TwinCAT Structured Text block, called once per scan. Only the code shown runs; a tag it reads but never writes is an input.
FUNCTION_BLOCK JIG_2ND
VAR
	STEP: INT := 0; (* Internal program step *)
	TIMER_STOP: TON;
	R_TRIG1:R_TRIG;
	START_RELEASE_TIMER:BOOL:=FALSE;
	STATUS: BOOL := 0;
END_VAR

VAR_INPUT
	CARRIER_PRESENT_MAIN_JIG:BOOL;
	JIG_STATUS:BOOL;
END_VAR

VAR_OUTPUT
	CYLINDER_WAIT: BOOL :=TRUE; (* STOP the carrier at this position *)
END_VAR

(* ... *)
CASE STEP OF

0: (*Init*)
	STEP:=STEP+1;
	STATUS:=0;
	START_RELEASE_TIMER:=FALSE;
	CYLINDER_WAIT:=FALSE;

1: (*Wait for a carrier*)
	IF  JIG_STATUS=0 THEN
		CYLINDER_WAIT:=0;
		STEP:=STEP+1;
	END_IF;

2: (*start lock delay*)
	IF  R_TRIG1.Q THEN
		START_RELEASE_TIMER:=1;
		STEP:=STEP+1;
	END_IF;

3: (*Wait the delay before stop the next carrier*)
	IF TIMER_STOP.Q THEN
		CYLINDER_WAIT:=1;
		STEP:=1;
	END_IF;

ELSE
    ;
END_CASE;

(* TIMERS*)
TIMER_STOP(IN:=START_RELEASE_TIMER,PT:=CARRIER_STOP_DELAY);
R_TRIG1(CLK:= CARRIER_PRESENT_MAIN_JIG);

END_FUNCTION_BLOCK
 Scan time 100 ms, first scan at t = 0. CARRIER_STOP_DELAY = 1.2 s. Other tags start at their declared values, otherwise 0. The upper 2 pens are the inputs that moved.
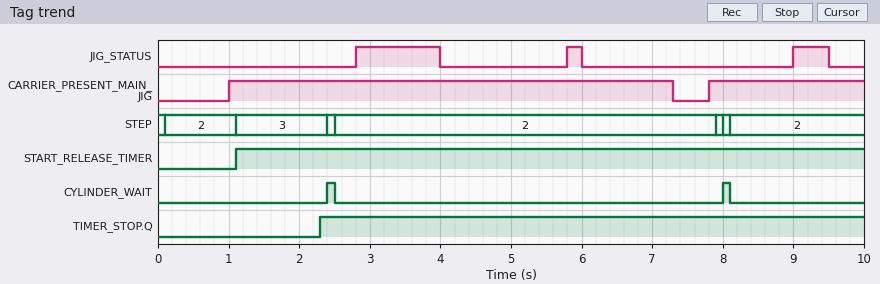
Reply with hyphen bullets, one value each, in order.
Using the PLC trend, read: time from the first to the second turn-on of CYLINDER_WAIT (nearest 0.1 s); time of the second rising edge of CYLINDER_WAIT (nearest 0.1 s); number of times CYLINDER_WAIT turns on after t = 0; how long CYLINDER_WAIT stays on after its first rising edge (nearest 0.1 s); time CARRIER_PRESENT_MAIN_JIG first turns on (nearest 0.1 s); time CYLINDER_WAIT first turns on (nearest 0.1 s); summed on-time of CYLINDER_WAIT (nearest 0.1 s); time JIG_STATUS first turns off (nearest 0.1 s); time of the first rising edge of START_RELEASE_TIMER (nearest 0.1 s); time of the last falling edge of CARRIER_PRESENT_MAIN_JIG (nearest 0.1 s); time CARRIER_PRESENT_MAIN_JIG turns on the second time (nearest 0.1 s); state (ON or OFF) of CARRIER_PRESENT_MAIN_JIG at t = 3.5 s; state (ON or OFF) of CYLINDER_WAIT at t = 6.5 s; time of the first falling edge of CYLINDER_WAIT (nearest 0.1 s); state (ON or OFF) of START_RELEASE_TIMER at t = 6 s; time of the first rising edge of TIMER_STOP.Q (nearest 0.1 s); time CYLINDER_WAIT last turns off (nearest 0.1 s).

- 5.6 s
- 8.0 s
- 2
- 0.1 s
- 1.0 s
- 2.4 s
- 0.2 s
- 4.0 s
- 1.1 s
- 7.3 s
- 7.8 s
- ON
- OFF
- 2.5 s
- ON
- 2.3 s
- 8.1 s
